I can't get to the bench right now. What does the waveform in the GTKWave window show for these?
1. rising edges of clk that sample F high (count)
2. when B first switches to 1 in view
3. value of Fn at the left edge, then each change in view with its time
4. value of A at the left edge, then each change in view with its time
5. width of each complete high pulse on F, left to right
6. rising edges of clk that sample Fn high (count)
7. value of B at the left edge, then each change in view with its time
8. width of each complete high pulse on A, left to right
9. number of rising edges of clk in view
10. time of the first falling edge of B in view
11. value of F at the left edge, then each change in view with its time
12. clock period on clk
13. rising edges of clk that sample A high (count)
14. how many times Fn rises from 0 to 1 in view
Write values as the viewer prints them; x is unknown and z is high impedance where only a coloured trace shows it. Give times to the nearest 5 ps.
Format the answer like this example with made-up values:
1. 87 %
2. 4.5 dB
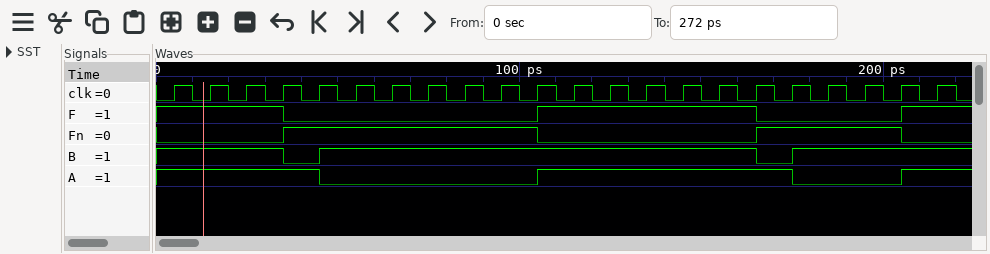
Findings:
1. 11
2. 45 ps
3. 0, 1 at 35 ps, 0 at 105 ps, 1 at 165 ps, 0 at 205 ps
4. 1, 0 at 45 ps, 1 at 105 ps, 0 at 175 ps, 1 at 205 ps
5. 60 ps
6. 11
7. 1, 0 at 35 ps, 1 at 45 ps, 0 at 165 ps, 1 at 175 ps
8. 70 ps
9. 22
10. 35 ps
11. 1, 0 at 35 ps, 1 at 105 ps, 0 at 165 ps, 1 at 205 ps
12. 10 ps
13. 13
14. 2
